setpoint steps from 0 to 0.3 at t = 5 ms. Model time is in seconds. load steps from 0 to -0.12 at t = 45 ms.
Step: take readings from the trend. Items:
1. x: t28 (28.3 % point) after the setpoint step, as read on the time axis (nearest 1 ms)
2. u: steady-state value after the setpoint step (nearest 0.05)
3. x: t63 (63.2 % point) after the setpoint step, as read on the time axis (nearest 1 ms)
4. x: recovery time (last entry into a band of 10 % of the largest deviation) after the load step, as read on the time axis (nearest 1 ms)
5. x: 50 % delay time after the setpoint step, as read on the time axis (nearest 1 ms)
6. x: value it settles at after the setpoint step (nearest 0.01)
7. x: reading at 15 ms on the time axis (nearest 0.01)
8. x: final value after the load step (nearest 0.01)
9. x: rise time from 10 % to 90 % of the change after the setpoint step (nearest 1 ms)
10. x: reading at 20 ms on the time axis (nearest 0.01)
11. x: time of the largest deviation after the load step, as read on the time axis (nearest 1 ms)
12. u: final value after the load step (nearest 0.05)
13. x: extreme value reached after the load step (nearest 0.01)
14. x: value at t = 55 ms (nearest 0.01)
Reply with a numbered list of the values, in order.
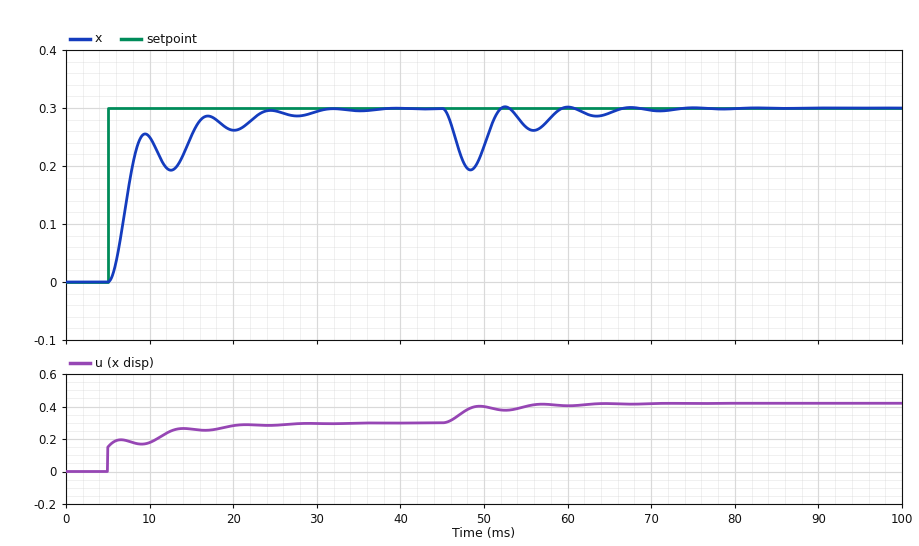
1. 7 ms
2. 0.30
3. 8 ms
4. 65 ms
5. 7 ms
6. 0.30
7. 0.25
8. 0.30
9. 10 ms
10. 0.26
11. 48 ms
12. 0.40
13. 0.19
14. 0.27
